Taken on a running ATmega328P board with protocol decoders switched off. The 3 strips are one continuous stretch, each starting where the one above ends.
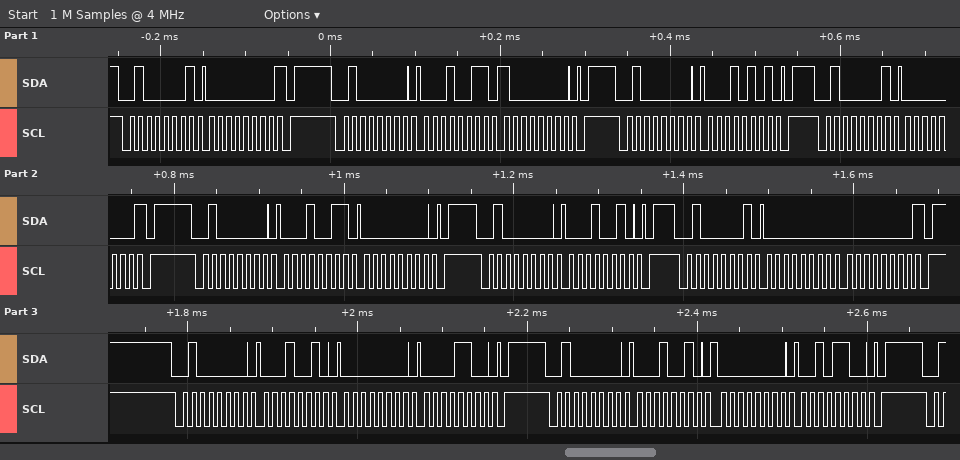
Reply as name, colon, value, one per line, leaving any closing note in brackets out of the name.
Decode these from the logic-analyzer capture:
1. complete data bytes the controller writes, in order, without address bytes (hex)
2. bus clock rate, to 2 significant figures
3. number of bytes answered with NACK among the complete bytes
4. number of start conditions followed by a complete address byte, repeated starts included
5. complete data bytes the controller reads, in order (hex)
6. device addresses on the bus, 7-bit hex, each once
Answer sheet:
complete data bytes the controller writes, in order, without address bytes: 13 80 15 13 00 12 12 00 0C 12 00 2C
bus clock rate, to 2 significant figures: 100 kHz
number of bytes answered with NACK among the complete bytes: 3
number of start conditions followed by a complete address byte, repeated starts included: 9
complete data bytes the controller reads, in order: 00 00 00 00
device addresses on the bus, 7-bit hex, each once: 0x20
